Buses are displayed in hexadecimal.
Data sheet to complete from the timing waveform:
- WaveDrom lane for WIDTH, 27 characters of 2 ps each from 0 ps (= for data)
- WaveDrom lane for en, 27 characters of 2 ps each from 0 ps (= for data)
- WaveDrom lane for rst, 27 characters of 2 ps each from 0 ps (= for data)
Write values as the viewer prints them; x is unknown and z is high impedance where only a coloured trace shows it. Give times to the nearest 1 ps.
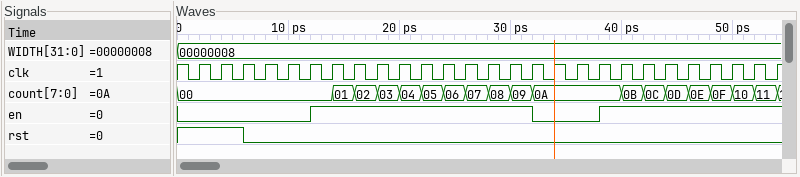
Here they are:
{name: 'WIDTH', wave: '=..........................', data: '00000008'}
{name: 'en', wave: '0.....1.........0..1.......'}
{name: 'rst', wave: '1..0.......................'}
